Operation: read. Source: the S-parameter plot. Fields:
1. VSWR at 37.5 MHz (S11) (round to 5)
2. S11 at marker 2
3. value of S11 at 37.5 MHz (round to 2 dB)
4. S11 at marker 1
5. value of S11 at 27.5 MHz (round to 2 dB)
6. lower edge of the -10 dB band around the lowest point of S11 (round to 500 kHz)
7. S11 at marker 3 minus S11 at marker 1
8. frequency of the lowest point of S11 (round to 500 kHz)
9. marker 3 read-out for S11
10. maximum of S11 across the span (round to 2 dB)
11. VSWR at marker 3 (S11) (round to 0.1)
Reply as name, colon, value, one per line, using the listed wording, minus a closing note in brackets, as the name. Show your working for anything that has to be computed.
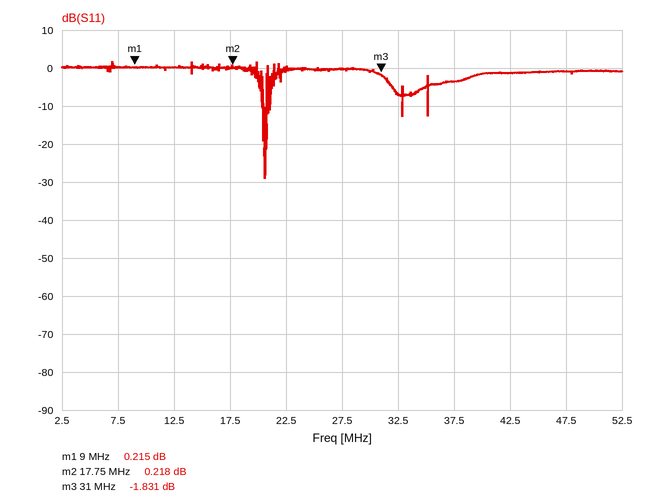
VSWR at 37.5 MHz (S11): |Γ| = 10^(-4/20) = 0.6310; VSWR = (1 + 0.6310)/(1 − 0.6310) ≈ 4.42, so 5 to the nearest 5
S11 at marker 2: 0.218 dB
value of S11 at 37.5 MHz: -4 dB
S11 at marker 1: 0.215 dB
value of S11 at 27.5 MHz: 0 dB
lower edge of the -10 dB band around the lowest point of S11: 20.5 MHz
S11 at marker 3 minus S11 at marker 1: -1.831 − (0.215) = -2.046 dB
frequency of the lowest point of S11: 20.5 MHz
marker 3 read-out for S11: -1.831 dB
maximum of S11 across the span: 2 dB
VSWR at marker 3 (S11): (1 + 0.8099)/(1 − 0.8099) ≈ 9.5
